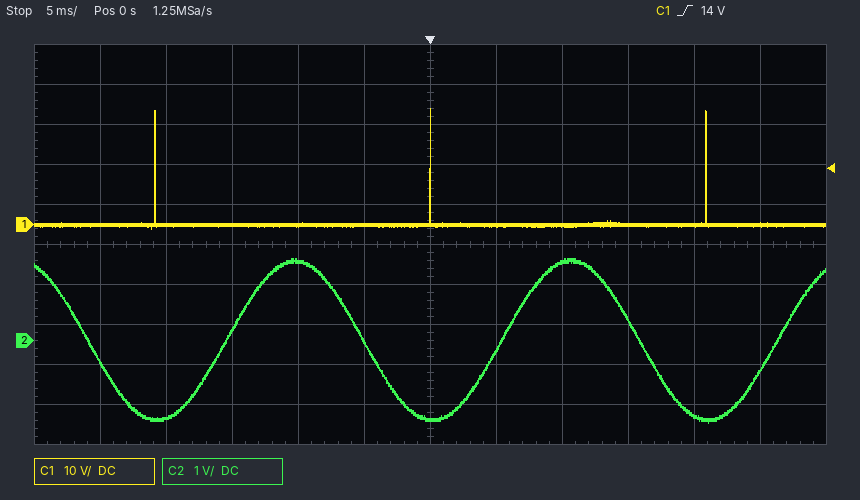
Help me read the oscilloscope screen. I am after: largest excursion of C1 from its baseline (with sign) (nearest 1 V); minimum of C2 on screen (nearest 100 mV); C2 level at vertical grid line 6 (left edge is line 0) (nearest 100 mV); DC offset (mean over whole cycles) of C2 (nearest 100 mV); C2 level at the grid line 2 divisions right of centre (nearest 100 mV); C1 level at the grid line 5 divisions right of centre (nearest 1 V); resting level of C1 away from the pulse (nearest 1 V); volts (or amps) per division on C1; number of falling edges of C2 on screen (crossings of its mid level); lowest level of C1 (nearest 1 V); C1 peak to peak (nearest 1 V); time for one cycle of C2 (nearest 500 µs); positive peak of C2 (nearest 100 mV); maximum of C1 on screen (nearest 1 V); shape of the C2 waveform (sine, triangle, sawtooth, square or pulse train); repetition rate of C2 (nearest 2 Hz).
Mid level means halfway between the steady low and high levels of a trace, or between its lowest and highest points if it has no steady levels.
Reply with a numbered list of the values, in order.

1. +29 V
2. -2.0 V
3. -2.0 V
4. 0.0 V
5. 2.0 V
6. 0 V
7. 0 V
8. 10 V
9. 3
10. -1 V
11. 30 V
12. 21.0 ms
13. 2.0 V
14. 29 V
15. sine
16. 48 Hz
